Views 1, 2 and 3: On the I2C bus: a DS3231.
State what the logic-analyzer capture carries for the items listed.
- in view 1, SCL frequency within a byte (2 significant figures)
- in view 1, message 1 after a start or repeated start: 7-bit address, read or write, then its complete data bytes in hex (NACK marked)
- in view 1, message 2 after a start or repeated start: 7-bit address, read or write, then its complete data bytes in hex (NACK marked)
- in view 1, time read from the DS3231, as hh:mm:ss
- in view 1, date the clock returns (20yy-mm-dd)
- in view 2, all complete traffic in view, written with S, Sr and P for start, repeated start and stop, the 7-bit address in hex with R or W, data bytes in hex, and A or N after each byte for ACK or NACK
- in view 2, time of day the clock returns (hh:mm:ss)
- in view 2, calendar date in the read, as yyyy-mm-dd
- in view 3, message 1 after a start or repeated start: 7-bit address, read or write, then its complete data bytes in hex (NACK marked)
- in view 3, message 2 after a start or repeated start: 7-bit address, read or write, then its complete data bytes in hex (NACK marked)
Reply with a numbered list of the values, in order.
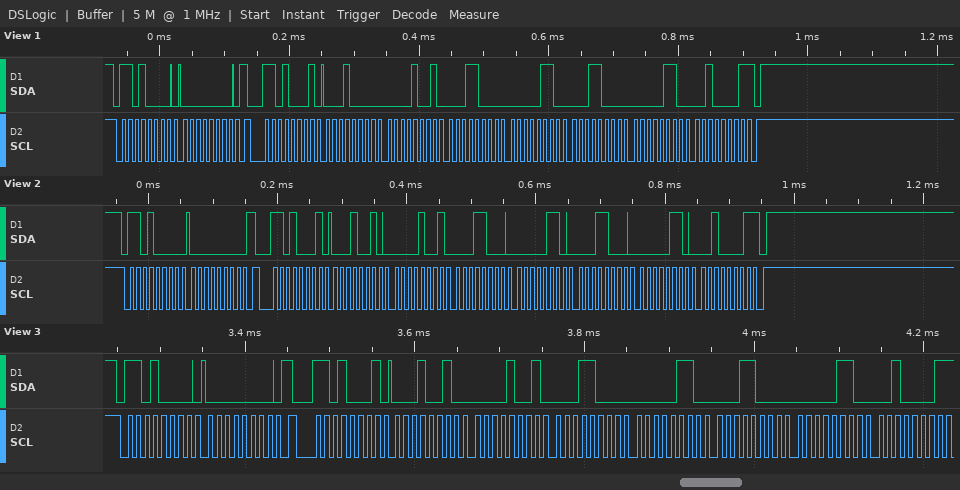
1. 100 kHz
2. 0x68 write: 00
3. 0x68 read: 10 09 18 06 18 06 21 NACK
4. 18:09:10
5. 2021-06-18
6. S 68W A 00 A Sr 68R A 12 A 09 A 18 A 06 A 18 A 06 A 21 N P
7. 18:09:12
8. 2021-06-18
9. 0x68 write: 00
10. 0x68 read: 12 09 18 06 18 06 21 NACK
